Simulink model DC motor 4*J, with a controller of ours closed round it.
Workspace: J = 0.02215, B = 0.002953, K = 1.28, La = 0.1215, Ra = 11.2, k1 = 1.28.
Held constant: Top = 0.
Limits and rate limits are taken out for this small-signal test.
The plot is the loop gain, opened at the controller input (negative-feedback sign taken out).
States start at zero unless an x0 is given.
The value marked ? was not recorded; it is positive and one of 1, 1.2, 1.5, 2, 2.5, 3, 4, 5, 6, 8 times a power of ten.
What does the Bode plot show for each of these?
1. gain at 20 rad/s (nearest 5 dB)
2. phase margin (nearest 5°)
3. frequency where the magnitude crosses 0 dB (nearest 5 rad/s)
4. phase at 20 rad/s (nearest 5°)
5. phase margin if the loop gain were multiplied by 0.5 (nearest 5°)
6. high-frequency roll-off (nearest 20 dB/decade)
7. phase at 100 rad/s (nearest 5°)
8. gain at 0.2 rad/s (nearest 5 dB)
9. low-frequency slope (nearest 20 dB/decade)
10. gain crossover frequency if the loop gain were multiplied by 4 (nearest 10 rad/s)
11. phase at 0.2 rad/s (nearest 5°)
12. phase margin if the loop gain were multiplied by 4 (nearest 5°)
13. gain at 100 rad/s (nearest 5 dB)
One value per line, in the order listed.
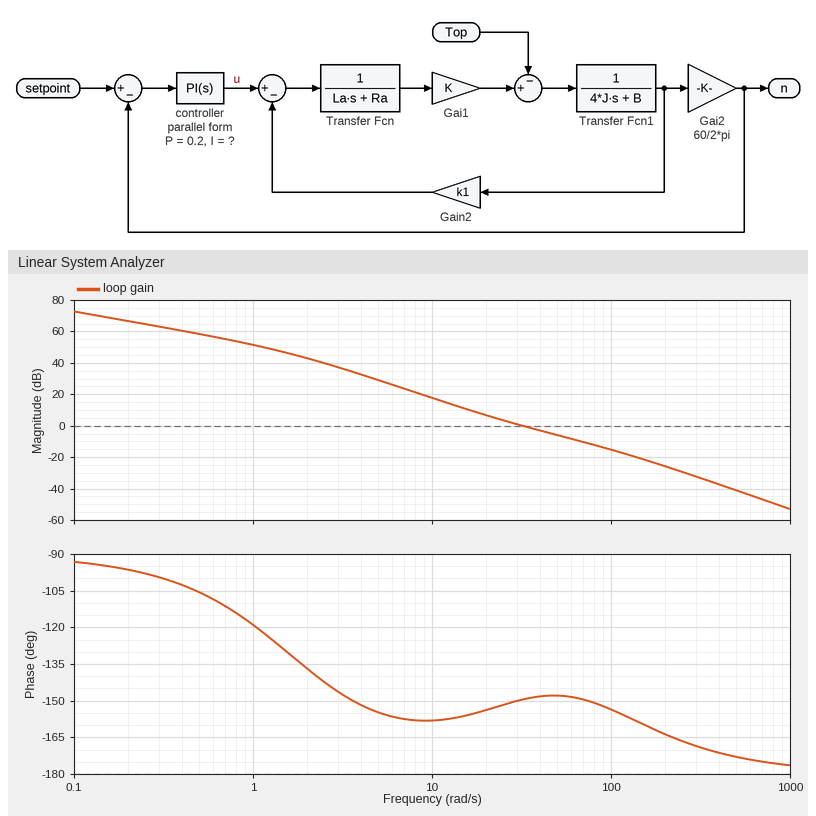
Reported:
5 dB
30°
30 rad/s
-155°
25°
-40 dB/decade
-155°
65 dB
-20 dB/decade
80 rad/s
-95°
30°
-15 dB
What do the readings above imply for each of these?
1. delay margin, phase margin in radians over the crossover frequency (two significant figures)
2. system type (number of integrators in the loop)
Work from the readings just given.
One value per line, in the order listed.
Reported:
0.017 s
1
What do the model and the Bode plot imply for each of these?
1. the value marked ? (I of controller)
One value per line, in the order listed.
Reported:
6
